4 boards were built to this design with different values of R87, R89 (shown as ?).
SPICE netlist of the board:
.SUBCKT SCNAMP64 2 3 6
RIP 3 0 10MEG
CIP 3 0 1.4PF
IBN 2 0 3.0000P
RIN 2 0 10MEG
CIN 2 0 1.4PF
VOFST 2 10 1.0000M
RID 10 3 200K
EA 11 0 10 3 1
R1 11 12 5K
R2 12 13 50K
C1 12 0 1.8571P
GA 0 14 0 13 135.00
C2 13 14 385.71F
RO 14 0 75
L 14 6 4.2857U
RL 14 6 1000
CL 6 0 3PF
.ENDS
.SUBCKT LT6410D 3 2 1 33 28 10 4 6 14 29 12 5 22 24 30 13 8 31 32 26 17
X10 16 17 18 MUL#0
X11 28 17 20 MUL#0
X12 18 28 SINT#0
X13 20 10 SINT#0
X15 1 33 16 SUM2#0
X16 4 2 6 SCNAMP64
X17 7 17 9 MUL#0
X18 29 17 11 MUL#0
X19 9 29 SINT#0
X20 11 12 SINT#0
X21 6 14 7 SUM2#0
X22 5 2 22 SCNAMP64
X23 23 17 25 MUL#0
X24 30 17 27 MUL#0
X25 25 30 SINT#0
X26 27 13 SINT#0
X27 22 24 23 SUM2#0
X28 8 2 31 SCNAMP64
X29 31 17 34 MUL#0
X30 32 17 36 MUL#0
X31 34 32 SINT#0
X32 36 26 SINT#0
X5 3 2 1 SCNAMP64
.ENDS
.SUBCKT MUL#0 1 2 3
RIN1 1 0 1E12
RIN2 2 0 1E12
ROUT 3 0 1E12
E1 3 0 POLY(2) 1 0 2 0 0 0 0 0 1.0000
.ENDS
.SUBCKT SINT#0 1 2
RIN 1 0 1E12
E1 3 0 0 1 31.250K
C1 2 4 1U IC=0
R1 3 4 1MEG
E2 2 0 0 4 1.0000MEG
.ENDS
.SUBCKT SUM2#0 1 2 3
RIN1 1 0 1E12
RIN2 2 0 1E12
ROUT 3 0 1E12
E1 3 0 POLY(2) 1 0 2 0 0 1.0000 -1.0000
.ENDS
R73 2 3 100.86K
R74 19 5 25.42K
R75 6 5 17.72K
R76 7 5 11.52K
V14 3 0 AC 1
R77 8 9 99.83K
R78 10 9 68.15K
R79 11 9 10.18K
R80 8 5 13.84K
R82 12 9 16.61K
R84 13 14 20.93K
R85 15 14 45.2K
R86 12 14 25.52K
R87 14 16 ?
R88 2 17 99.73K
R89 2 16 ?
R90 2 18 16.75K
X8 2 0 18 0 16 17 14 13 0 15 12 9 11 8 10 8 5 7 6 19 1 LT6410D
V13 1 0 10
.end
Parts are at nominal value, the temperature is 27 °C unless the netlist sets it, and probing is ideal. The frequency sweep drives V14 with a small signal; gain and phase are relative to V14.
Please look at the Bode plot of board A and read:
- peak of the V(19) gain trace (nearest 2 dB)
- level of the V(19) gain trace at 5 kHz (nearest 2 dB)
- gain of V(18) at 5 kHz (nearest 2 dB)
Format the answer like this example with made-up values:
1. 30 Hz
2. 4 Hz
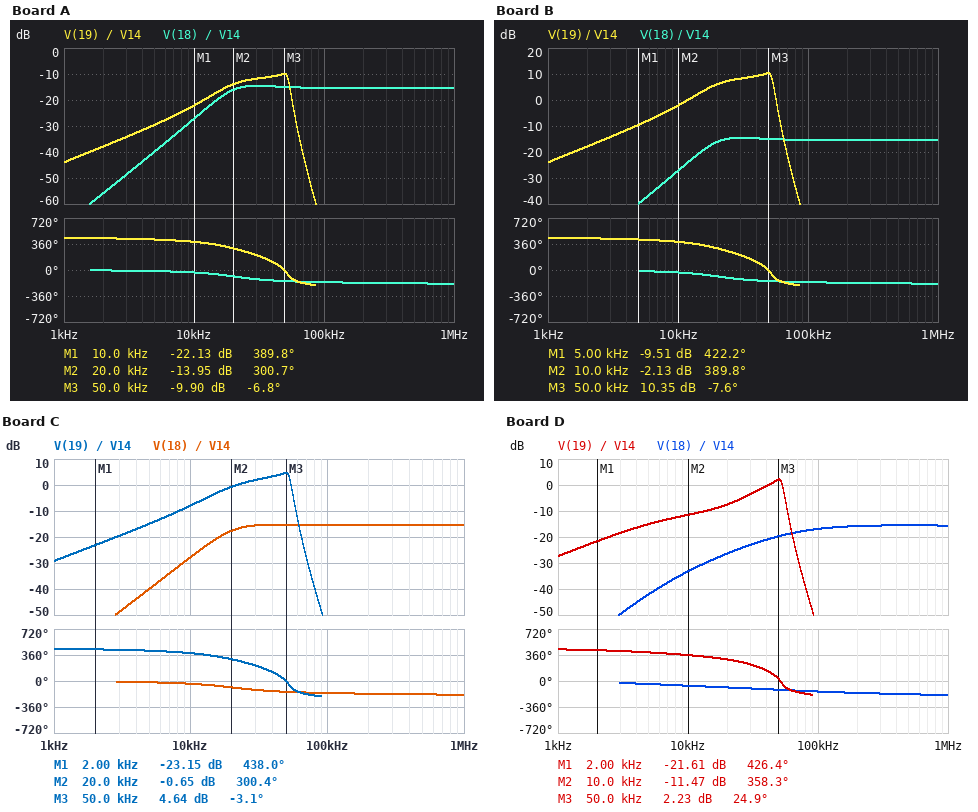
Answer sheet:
1. -10 dB
2. -30 dB
3. -40 dB
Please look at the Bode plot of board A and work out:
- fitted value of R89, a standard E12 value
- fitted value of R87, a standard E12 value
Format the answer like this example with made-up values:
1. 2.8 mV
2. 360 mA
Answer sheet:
1. 39 kΩ
2. 82 kΩ
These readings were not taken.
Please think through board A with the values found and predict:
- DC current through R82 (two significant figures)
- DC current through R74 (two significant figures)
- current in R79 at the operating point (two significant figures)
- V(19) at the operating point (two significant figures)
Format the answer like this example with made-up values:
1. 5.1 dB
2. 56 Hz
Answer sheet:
1. 130 nA
2. 220 nA
3. 100 nA
4. 6.5 mV
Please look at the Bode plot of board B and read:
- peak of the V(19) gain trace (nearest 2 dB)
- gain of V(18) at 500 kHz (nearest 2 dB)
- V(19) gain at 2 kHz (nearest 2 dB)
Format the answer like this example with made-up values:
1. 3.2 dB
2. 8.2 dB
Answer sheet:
1. 10 dB
2. -16 dB
3. -18 dB
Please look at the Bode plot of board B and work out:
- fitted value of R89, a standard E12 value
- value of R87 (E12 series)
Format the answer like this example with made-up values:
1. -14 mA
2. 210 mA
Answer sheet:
1. 39 kΩ
2. 8.2 kΩ
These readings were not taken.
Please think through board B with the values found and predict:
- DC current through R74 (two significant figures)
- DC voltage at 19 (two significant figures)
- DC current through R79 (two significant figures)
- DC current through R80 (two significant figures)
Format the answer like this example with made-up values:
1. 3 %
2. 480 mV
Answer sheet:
1. 330 nA
2. 9.4 mV
3. 250 nA
4. 190 nA
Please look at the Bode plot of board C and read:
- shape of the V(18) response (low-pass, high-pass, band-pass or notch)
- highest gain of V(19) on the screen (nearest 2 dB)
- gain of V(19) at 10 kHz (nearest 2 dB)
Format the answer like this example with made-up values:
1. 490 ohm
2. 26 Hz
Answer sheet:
1. high-pass
2. 4 dB
3. -8 dB
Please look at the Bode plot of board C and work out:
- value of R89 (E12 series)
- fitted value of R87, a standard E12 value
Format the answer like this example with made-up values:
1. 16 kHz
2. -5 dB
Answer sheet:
1. 33 kΩ
2. 15 kΩ
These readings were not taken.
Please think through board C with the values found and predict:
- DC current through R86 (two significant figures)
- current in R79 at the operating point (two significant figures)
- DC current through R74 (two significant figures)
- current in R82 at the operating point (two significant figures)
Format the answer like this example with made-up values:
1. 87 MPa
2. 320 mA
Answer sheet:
1. 140 nA
2. 180 nA
3. 270 nA
4. 210 nA
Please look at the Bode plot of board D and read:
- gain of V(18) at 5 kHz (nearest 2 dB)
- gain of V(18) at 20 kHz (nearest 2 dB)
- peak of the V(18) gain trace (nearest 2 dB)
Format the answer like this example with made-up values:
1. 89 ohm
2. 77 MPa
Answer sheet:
1. -42 dB
2. -26 dB
3. -16 dB
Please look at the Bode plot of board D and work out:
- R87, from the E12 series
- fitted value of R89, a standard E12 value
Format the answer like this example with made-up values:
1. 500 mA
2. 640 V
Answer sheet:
1. 12 kΩ
2. 12 kΩ
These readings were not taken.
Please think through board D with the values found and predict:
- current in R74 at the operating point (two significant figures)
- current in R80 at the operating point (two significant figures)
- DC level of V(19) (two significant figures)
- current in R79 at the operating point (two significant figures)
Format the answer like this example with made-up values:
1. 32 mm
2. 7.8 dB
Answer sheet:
1. 290 nA
2. 150 nA
3. 8.4 mV
4. 200 nA
